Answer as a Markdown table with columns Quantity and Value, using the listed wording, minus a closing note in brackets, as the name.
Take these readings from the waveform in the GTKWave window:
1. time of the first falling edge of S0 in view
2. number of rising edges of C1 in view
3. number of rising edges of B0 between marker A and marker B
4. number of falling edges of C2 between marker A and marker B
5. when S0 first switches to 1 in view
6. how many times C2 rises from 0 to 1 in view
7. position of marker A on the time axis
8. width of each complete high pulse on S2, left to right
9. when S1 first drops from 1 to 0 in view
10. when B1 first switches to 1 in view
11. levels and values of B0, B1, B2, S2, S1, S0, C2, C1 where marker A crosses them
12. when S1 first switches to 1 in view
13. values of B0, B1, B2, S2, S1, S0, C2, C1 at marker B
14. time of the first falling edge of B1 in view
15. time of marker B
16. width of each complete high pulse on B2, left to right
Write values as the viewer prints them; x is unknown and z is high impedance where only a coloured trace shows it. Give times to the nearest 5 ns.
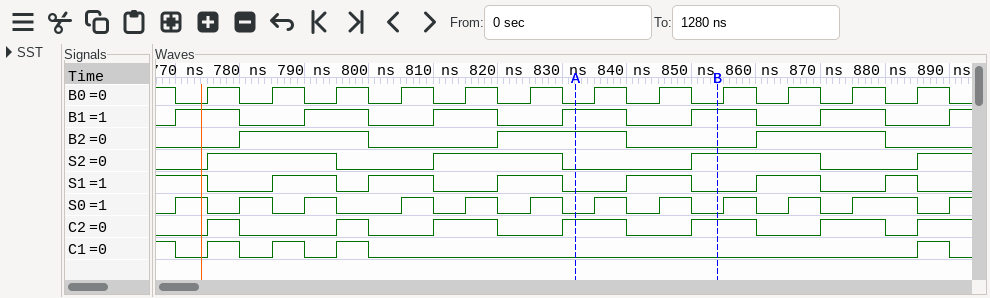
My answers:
| Quantity | Value |
|---|---|
| time of the first falling edge of S0 in view | 775 ns |
| number of rising edges of C1 in view | 4 |
| number of rising edges of B0 between marker A and marker B | 2 |
| number of falling edges of C2 between marker A and marker B | 1 |
| when S0 first switches to 1 in view | 770 ns |
| how many times C2 rises from 0 to 1 in view | 7 |
| position of marker A on the time axis | 830 ns |
| width of each complete high pulse on S2, left to right | 20 ns, 20 ns, 20 ns |
| when S1 first drops from 1 to 0 in view | 775 ns |
| when B1 first switches to 1 in view | 770 ns |
| levels and values of B0, B1, B2, S2, S1, S0, C2, C1 where marker A crosses them | B0=0, B1=1, B2=1, S2=0, S1=0, S0=0, C2=1, C1=0 |
| when S1 first switches to 1 in view | 785 ns |
| values of B0, B1, B2, S2, S1, S0, C2, C1 at marker B | B0=0, B1=1, B2=0, S2=1, S1=0, S0=0, C2=1, C1=0 |
| time of the first falling edge of B1 in view | 780 ns |
| time of marker B | 855 ns |
| width of each complete high pulse on B2, left to right | 20 ns, 20 ns, 20 ns |
